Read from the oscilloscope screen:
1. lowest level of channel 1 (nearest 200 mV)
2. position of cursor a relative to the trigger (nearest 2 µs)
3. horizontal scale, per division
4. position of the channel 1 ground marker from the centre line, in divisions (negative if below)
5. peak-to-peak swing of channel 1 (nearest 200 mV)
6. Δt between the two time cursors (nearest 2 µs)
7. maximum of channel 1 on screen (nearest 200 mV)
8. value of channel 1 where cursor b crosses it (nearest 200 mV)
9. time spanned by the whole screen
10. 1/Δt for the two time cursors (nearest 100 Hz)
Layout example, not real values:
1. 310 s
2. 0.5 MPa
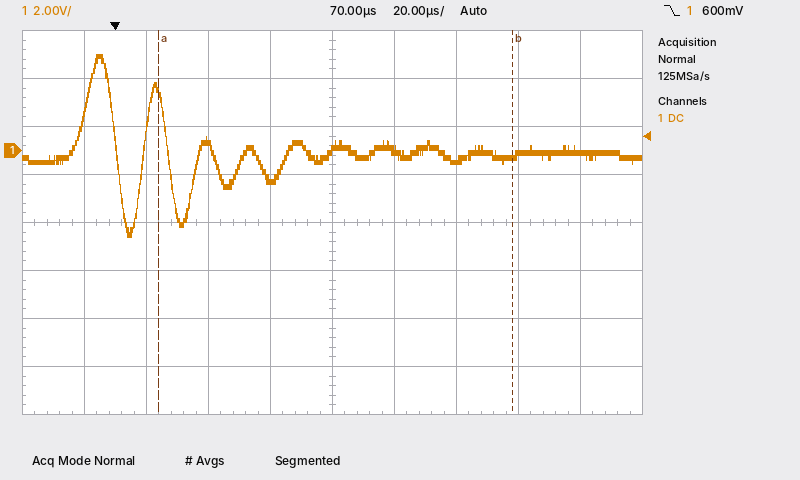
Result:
1. -3.6 V
2. +14 µs
3. 20 µs
4. +1.5 div
5. 7.6 V
6. 114 µs
7. 4.0 V
8. -200 mV
9. 200 µs
10. 8.8 kHz
